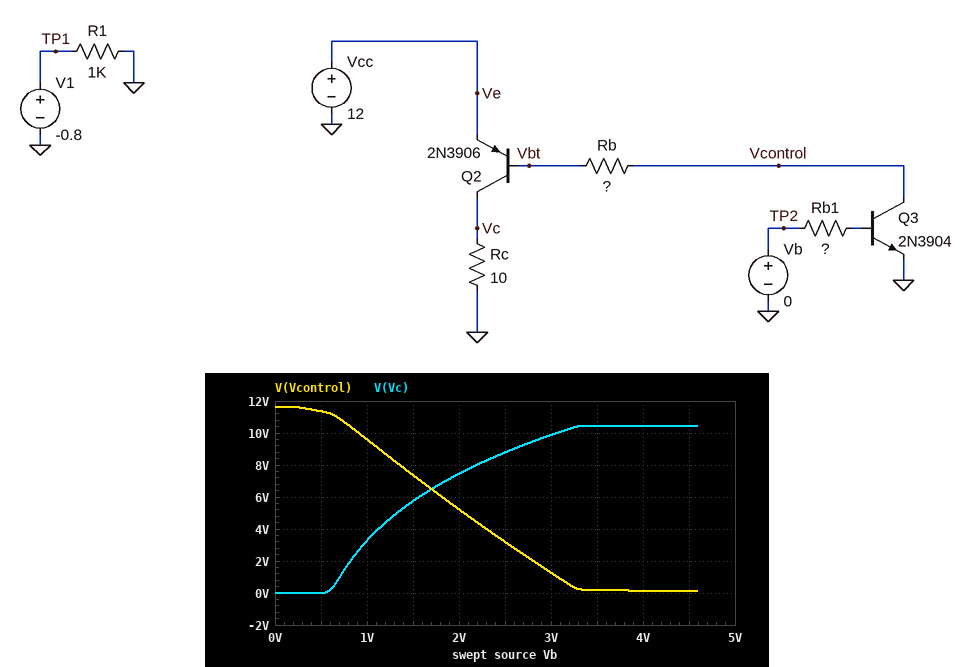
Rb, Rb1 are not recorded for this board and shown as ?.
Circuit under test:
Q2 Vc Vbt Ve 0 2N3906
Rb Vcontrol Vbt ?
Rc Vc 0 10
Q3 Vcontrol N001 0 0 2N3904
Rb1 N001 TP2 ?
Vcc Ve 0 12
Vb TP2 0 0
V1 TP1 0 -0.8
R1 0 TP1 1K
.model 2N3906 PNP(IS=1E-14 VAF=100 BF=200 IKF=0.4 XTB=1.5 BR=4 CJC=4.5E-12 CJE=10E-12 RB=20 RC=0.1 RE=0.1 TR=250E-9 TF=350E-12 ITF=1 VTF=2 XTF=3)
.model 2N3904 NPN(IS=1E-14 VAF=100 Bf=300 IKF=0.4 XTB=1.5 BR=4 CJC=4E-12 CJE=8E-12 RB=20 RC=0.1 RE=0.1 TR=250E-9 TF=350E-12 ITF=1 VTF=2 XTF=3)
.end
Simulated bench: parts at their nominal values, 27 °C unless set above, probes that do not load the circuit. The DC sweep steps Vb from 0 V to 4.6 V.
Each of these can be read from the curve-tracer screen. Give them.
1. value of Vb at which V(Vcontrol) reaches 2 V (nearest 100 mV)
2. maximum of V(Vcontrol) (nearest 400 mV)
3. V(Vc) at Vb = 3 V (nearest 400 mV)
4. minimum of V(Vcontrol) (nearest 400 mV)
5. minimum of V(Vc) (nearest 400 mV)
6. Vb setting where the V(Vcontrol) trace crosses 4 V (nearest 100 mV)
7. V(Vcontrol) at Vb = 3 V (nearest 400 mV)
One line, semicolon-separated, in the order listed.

2.8 V; 11.6 V; 10.0 V; 0 V; 0 V; 2.3 V; 1.2 V
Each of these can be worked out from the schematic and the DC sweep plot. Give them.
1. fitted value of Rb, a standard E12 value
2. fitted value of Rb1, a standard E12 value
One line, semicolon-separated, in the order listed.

560 Ω; 39 kΩ
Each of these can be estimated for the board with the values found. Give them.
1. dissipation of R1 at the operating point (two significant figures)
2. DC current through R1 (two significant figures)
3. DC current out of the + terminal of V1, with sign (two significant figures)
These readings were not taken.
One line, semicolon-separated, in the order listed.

640 µW; 800 µA; -800 µA
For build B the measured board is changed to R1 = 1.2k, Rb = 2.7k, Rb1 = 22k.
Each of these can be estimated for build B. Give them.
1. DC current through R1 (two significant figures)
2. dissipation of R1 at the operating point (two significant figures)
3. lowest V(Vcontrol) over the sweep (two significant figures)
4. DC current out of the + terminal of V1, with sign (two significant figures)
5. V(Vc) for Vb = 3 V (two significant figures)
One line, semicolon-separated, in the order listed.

670 µA; 530 µW; 54 mV; -670 µA; 4.3 V
